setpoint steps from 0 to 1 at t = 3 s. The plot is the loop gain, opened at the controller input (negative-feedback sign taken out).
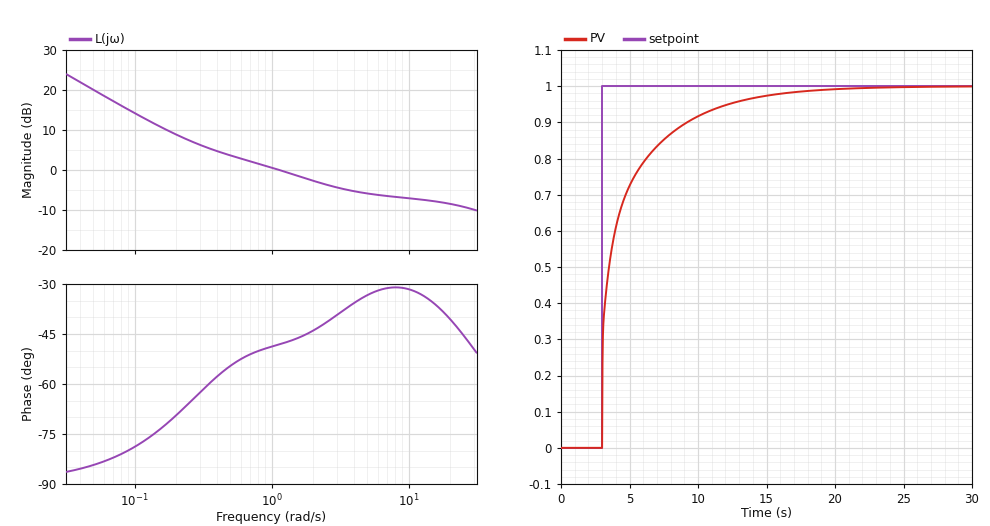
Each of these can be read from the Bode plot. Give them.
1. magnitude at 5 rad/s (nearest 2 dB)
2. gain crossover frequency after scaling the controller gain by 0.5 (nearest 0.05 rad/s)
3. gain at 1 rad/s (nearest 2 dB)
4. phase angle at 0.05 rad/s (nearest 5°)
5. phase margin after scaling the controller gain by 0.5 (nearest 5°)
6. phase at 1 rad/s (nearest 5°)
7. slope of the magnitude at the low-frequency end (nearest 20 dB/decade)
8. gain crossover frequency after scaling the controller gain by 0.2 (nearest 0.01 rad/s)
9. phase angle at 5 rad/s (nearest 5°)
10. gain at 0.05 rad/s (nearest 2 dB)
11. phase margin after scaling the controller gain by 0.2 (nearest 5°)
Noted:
-6 dB
0.30 rad/s
0 dB
-85°
120°
-50°
-20 dB/decade
0.10 rad/s
-35°
20 dB
100°
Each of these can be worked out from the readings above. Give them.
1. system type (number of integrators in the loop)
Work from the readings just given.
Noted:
1
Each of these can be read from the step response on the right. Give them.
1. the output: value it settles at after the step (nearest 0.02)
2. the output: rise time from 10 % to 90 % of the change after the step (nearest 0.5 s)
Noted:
1.00
6.0 s
